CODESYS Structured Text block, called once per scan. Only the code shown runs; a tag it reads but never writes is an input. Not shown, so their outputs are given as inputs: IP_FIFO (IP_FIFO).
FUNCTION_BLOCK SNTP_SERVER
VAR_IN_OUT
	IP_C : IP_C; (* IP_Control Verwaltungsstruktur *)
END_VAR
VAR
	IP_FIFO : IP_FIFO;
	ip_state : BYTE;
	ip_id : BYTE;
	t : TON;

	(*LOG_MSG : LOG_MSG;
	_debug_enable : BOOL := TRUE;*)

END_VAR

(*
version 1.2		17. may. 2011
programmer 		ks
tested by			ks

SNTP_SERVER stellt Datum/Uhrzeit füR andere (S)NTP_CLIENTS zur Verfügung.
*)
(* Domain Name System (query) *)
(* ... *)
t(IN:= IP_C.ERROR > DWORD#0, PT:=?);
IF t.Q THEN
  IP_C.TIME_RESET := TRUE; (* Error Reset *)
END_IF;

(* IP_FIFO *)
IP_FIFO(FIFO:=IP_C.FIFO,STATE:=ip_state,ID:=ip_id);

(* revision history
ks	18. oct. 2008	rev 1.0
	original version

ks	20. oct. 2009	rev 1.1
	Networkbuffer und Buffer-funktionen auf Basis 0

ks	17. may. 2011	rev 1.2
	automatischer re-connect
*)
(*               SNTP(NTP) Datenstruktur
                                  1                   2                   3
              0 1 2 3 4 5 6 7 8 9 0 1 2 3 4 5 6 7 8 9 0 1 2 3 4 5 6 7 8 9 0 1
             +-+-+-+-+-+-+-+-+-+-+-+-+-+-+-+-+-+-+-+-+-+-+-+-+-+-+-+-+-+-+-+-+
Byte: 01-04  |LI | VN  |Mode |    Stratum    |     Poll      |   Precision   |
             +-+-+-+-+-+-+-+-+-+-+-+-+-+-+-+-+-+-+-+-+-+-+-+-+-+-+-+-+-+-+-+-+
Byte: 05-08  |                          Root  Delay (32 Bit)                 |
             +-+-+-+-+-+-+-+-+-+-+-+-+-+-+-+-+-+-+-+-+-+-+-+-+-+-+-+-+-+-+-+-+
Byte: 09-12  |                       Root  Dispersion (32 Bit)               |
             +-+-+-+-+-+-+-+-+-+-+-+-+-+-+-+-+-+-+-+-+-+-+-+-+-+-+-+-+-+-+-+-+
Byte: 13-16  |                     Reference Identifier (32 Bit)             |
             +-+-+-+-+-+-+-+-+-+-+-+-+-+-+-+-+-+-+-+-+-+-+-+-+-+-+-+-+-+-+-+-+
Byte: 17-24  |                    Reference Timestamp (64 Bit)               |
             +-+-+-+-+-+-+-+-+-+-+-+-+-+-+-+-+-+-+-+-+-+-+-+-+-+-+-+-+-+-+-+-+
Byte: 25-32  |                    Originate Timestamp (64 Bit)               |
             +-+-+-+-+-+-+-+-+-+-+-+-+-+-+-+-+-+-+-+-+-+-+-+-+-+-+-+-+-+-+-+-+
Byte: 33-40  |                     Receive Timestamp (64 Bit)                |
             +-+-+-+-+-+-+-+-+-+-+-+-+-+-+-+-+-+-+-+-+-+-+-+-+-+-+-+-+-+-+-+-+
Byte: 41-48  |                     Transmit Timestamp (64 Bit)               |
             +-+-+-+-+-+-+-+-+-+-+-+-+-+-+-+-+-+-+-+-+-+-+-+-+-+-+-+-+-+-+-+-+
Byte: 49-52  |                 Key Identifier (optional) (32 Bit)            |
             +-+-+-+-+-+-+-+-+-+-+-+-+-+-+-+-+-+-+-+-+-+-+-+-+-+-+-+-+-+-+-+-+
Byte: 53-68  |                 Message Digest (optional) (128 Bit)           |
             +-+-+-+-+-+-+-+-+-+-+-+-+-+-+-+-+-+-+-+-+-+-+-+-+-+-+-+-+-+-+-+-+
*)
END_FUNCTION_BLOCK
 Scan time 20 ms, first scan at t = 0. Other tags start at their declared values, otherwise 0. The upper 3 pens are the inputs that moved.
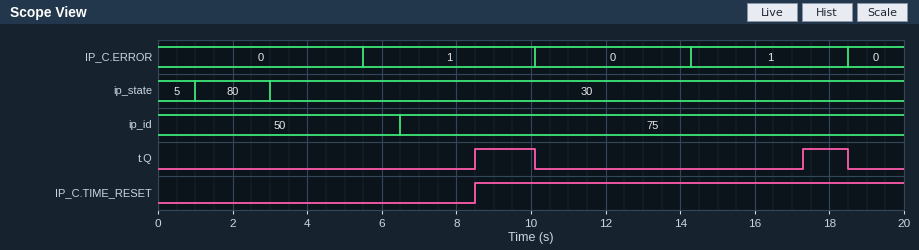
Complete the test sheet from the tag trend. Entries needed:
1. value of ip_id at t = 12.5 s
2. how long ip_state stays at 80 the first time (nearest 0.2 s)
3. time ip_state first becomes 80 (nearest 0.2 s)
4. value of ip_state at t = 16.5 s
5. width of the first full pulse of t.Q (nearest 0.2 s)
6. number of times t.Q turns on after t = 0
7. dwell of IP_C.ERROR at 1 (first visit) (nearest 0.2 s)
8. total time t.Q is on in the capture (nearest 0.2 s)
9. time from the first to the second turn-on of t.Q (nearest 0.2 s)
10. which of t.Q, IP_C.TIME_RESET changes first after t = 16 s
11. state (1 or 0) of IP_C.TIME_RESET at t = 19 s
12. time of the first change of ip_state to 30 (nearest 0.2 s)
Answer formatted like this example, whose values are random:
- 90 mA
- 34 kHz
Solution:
- 75
- 2.0 s
- 1.0 s
- 30
- 1.6 s
- 2
- 4.6 s
- 2.8 s
- 8.8 s
- t.Q
- 1
- 3.0 s
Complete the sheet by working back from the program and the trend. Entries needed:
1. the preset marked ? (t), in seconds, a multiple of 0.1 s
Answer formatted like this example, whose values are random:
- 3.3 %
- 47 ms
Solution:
- 3.0 s
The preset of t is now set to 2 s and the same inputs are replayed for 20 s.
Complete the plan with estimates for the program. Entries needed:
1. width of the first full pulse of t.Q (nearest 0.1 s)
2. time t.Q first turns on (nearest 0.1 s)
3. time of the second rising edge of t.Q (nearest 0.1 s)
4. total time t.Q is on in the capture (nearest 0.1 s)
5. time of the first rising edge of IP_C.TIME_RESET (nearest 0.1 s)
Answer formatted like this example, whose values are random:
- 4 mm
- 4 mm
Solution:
- 2.6 s
- 7.5 s
- 16.3 s
- 4.8 s
- 7.5 s
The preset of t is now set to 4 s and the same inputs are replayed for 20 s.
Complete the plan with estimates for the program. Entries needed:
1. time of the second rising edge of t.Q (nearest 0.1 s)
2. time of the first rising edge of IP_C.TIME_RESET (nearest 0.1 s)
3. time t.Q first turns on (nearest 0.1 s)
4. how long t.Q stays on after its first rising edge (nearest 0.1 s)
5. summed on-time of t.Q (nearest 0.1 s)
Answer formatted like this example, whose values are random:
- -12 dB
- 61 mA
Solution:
- 18.3 s
- 9.5 s
- 9.5 s
- 0.6 s
- 0.8 s
